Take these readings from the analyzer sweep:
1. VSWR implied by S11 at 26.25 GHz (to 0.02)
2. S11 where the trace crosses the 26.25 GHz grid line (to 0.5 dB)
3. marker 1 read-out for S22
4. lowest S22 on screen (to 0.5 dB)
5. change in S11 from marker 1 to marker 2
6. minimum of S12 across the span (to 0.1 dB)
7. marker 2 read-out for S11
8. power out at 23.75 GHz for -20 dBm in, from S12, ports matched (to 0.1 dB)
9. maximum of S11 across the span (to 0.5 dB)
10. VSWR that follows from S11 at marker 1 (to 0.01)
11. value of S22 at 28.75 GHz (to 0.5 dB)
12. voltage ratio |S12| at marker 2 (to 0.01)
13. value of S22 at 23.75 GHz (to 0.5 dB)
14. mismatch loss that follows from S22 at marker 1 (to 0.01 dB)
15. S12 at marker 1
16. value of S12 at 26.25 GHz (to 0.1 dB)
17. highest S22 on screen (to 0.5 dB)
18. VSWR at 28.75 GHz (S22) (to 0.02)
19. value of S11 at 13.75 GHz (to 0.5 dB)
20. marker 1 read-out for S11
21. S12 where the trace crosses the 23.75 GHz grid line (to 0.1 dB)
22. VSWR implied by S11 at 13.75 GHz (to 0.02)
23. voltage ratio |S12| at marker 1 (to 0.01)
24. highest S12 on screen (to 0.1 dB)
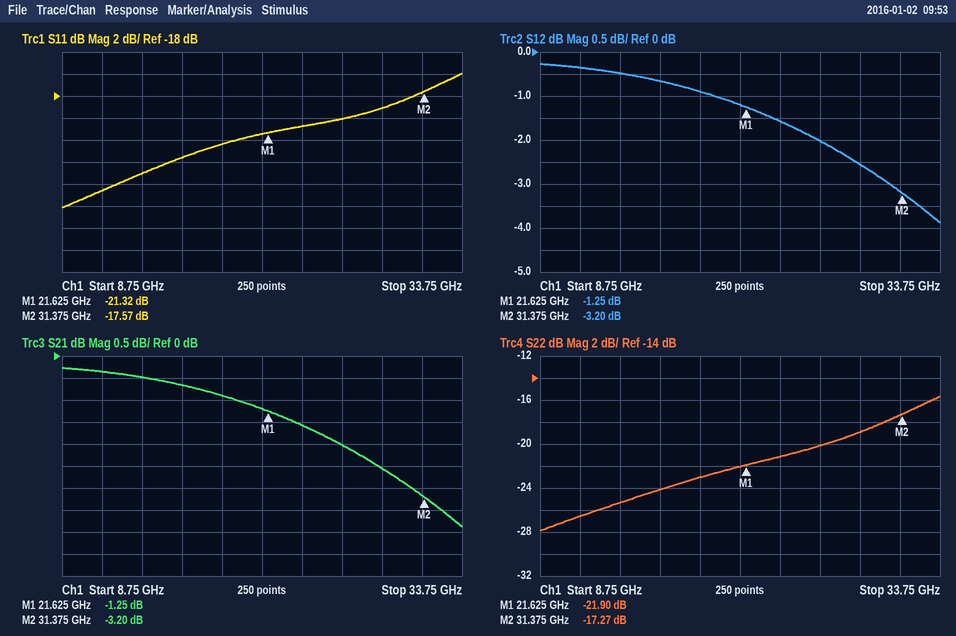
1.22
-20.0 dB
-21.90 dB
-28.0 dB
3.75 dB
-3.9 dB
-17.57 dB
-21.6 dBm
-16.0 dB
1.19
-19.0 dB
0.69
-21.0 dB
0.03 dB
-1.25 dB
-2.0 dB
-15.5 dB
1.26
-25.0 dB
-21.32 dB
-1.6 dB
1.12
0.87
-0.3 dB
